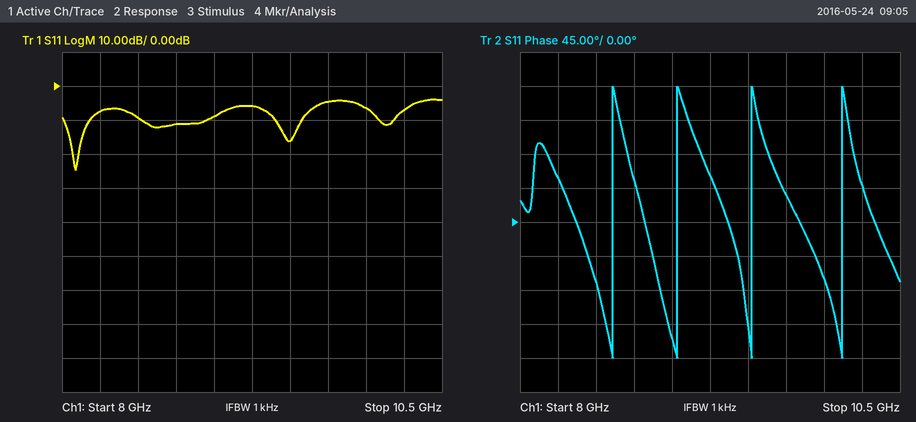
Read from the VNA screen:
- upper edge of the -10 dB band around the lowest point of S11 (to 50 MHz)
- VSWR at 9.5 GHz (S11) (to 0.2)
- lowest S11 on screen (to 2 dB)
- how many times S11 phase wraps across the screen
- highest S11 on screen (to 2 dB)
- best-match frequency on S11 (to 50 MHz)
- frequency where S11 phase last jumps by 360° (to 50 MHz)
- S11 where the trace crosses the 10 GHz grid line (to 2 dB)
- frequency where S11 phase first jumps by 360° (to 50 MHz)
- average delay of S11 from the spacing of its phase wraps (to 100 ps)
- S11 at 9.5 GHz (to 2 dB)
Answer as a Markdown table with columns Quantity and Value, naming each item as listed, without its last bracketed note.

| Quantity | Value |
|---|---|
| upper edge of the -10 dB band around the lowest point of S11 | 8.20 GHz |
| VSWR at 9.5 GHz (S11) | 1.4 |
| lowest S11 on screen | -24 dB |
| how many times S11 phase wraps across the screen | 4 |
| highest S11 on screen | -4 dB |
| best-match frequency on S11 | 8.10 GHz |
| frequency where S11 phase last jumps by 360° | 10.10 GHz |
| S11 where the trace crosses the 10 GHz grid line | -6 dB |
| frequency where S11 phase first jumps by 360° | 8.60 GHz |
| average delay of S11 from the spacing of its phase wraps | 2.0 ns |
| S11 at 9.5 GHz | -16 dB |
